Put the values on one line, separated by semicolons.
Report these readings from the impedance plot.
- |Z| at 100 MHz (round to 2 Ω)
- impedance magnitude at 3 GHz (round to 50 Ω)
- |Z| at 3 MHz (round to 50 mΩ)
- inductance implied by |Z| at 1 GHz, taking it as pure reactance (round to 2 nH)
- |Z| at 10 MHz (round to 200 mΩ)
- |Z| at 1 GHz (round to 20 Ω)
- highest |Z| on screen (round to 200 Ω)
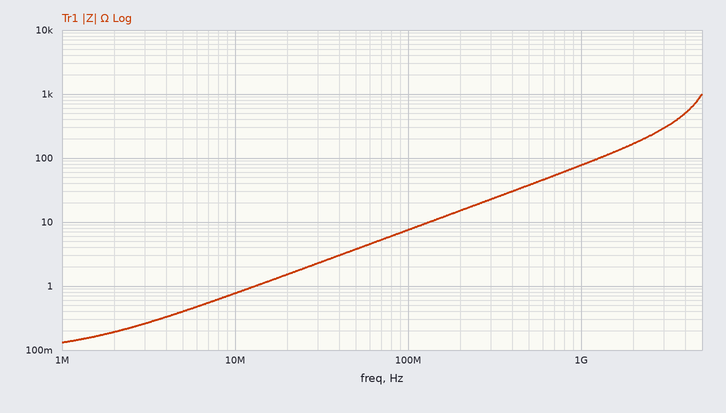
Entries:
8 Ω; 300 Ω; 250 mΩ; 12 nH; 800 mΩ; 80 Ω; 1.0 kΩ
